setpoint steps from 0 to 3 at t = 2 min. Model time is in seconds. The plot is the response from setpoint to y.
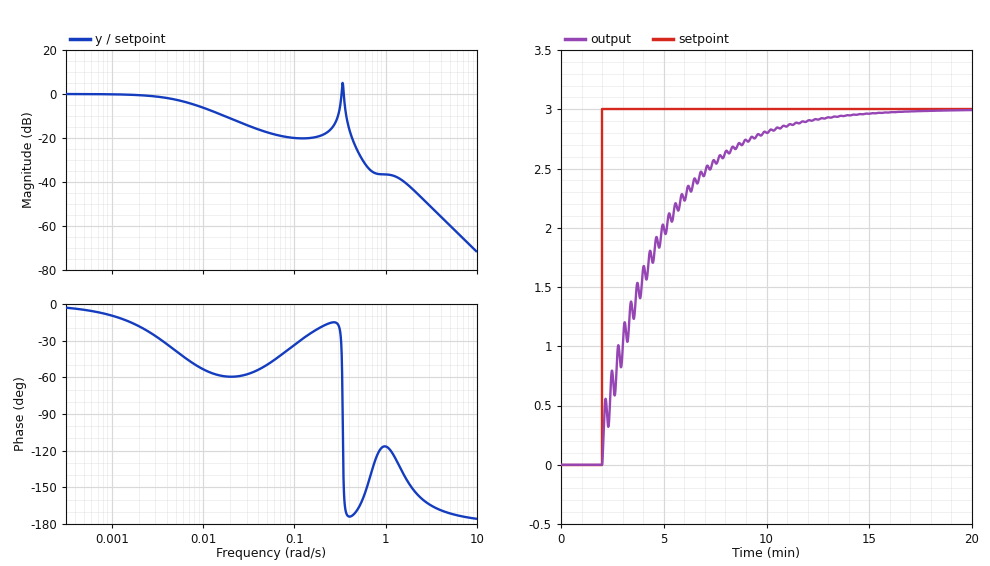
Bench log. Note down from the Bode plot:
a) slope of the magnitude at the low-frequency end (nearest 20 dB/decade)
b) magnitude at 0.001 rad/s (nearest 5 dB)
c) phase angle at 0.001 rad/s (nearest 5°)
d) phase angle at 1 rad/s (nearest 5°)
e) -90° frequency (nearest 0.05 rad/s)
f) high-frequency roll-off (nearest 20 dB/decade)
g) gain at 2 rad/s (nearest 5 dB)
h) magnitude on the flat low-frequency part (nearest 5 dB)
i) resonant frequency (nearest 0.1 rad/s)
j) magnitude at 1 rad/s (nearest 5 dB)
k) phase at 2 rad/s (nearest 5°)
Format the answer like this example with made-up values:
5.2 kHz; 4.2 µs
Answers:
0 dB/decade; 0 dB; -10°; -115°; 0.35 rad/s; -40 dB/decade; -45 dB; 0 dB; 0.3 rad/s; -35 dB; -150°
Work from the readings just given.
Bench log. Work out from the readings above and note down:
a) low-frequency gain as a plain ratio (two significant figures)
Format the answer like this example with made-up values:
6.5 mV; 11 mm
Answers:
1.0
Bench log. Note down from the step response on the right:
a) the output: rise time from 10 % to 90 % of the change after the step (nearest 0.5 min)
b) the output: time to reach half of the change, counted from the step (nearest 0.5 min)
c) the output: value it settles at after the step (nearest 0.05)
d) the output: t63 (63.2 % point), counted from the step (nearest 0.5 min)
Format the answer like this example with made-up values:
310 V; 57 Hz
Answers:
6.5 min; 1.5 min; 3.00; 2.5 min
